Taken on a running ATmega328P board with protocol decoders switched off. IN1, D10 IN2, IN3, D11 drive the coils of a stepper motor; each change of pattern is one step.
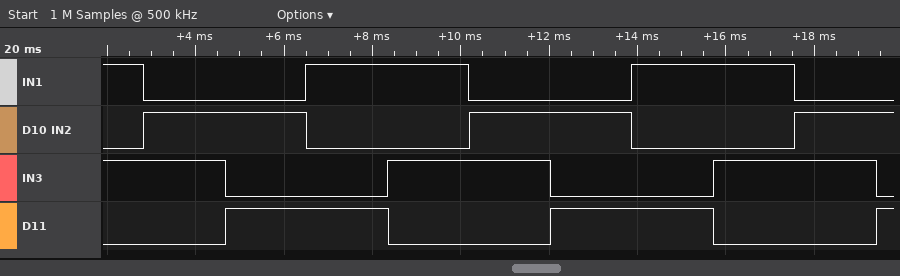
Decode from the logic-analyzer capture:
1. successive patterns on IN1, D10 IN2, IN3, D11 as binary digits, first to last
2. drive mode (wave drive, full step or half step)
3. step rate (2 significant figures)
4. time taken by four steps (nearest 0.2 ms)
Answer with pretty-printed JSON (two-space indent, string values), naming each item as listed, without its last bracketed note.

{
  "successive patterns on IN1, D10 IN2, IN3, D11 as binary digits, first to last": "1010 0110 0101 1001 1010 0110 0101 1001 1010 0110 0101",
  "drive mode": "full step",
  "step rate": "540 steps/s",
  "time taken by four steps": "7.4 ms"
}
